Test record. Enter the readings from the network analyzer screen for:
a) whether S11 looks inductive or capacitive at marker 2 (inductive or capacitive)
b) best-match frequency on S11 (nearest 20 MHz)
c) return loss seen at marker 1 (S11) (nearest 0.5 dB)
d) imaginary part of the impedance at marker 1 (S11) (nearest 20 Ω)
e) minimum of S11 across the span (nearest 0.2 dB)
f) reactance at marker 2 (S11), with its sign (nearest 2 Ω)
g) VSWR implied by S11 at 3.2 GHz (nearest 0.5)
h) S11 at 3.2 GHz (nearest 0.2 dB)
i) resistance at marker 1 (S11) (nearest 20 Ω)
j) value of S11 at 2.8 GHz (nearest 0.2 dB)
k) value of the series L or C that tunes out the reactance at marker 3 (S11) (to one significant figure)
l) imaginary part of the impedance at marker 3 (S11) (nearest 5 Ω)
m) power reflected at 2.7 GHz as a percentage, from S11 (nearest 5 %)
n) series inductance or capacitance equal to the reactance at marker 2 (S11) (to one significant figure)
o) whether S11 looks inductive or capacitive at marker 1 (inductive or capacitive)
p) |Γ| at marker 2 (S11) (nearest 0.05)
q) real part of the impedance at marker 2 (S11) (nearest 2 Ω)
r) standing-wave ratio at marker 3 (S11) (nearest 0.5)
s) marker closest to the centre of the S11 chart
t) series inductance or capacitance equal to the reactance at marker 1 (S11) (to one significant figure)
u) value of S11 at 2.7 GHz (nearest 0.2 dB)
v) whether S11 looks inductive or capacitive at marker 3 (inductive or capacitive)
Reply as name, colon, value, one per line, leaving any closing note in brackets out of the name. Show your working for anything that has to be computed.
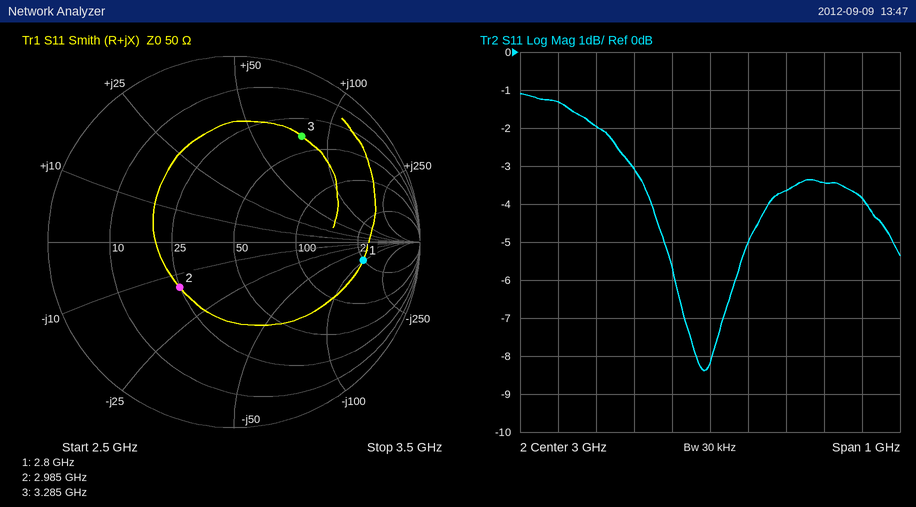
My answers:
whether S11 looks inductive or capacitive at marker 2: capacitive
best-match frequency on S11: 2.98 GHz
return loss seen at marker 1 (S11): 3.0 dB
imaginary part of the impedance at marker 1 (S11): -100 Ω
minimum of S11 across the span: -8.4 dB
reactance at marker 2 (S11), with its sign: -14 Ω
VSWR implied by S11 at 3.2 GHz: |Γ| = 10^(-3.6/20) = 0.6607; VSWR = (1 + 0.6607)/(1 − 0.6607) ≈ 4.89, so 5.0 to the nearest 0.5
S11 at 3.2 GHz: -3.6 dB
resistance at marker 1 (S11): 240 Ω
value of S11 at 2.8 GHz: -3.0 dB
value of the series L or C that tunes out the reactance at marker 3 (S11): C = 1/(2π × 3.285 GHz × 80 Ω) ≈ 606 fF, so 600 fF to one significant figure
imaginary part of the impedance at marker 3 (S11): +80 Ω
power reflected at 2.7 GHz as a percentage, from S11: 10^(-2/10) ≈ 63.1 %, so 65 % to the nearest 5 %
series inductance or capacitance equal to the reactance at marker 2 (S11): C = 1/(2π × 2.985 GHz × 14 Ω) ≈ 4 pF
whether S11 looks inductive or capacitive at marker 1: capacitive
|Γ| at marker 2 (S11): 0.40
real part of the impedance at marker 2 (S11): 24 Ω
standing-wave ratio at marker 3 (S11): 5.0
marker closest to the centre of the S11 chart: marker 2
series inductance or capacitance equal to the reactance at marker 1 (S11): C = 1/(2π × 2.8 GHz × 100 Ω) ≈ 568 fF, so 600 fF to one significant figure
value of S11 at 2.7 GHz: -2.0 dB
whether S11 looks inductive or capacitive at marker 3: inductive
